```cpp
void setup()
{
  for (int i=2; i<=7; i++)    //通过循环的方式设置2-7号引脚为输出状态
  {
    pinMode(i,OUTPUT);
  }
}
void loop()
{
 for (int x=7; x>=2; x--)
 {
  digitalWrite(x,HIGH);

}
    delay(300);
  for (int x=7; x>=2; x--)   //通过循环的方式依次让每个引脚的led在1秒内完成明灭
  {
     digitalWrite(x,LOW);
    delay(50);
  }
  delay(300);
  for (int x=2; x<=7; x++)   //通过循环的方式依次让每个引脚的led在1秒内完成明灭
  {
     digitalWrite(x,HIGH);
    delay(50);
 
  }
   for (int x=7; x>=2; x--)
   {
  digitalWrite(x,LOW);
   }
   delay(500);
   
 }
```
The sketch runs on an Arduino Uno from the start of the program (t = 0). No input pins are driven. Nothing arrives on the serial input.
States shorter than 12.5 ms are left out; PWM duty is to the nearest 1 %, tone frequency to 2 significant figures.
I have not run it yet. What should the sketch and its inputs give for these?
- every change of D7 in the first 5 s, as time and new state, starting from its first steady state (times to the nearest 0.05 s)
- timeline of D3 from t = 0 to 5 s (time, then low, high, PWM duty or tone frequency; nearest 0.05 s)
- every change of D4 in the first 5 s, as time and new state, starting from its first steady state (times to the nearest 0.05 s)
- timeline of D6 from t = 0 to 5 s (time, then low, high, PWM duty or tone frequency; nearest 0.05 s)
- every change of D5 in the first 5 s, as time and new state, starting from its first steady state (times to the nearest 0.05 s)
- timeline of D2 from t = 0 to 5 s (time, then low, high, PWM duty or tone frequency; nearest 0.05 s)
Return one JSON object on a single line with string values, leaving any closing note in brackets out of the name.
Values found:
{"every change of D7 in the first 5 s, as time and new state, starting from its first steady state": "0 s high; 0.3 s low; 1.15 s high; 1.2 s low; 1.7 s high; 2 s low; 2.85 s high; 2.9 s low; 3.4 s high; 3.7 s low; 4.55 s high; 4.6 s low", "timeline of D3 from t = 0 to 5 s": "0 s high; 0.5 s low; 0.95 s high; 1.2 s low; 1.7 s high; 2.2 s low; 2.65 s high; 2.9 s low; 3.4 s high; 3.9 s low; 4.35 s high; 4.6 s low", "every change of D4 in the first 5 s, as time and new state, starting from its first steady state": "0 s high; 0.45 s low; 1 s high; 1.2 s low; 1.7 s high; 2.15 s low; 2.7 s high; 2.9 s low; 3.4 s high; 3.85 s low; 4.4 s high; 4.6 s low", "timeline of D6 from t = 0 to 5 s": "0 s high; 0.35 s low; 1.1 s high; 1.2 s low; 1.7 s high; 2.05 s low; 2.8 s high; 2.9 s low; 3.4 s high; 3.75 s low; 4.5 s high; 4.6 s low", "every change of D5 in the first 5 s, as time and new state, starting from its first steady state": "0 s high; 0.4 s low; 1.05 s high; 1.2 s low; 1.7 s high; 2.1 s low; 2.75 s high; 2.9 s low; 3.4 s high; 3.8 s low; 4.45 s high; 4.6 s low", "timeline of D2 from t = 0 to 5 s": "0 s high; 0.55 s low; 0.9 s high; 1.2 s low; 1.7 s high; 2.25 s low; 2.6 s high; 2.9 s low; 3.4 s high; 3.95 s low; 4.3 s high; 4.6 s low"}
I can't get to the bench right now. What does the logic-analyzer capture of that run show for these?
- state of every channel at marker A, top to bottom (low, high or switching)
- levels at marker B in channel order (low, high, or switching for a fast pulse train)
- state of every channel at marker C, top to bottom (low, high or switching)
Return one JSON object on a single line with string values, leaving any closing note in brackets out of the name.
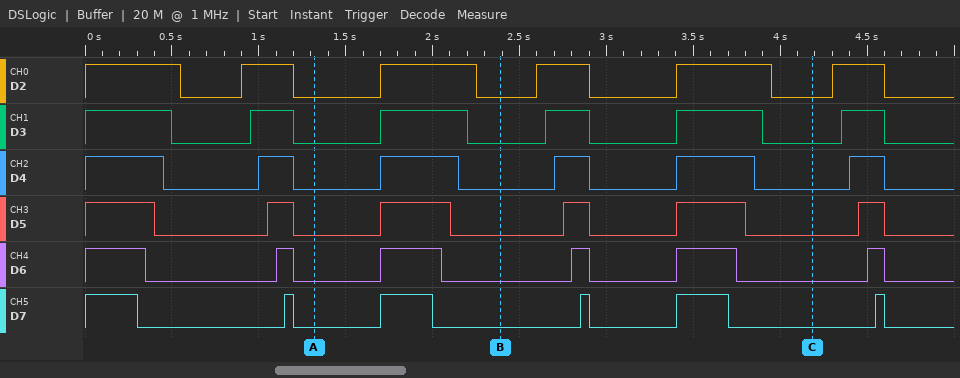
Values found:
{"state of every channel at marker A, top to bottom": "D2 low, D3 low, D4 low, D5 low, D6 low, D7 low", "levels at marker B in channel order": "D2 low, D3 low, D4 low, D5 low, D6 low, D7 low", "state of every channel at marker C, top to bottom": "D2 low, D3 low, D4 low, D5 low, D6 low, D7 low"}
